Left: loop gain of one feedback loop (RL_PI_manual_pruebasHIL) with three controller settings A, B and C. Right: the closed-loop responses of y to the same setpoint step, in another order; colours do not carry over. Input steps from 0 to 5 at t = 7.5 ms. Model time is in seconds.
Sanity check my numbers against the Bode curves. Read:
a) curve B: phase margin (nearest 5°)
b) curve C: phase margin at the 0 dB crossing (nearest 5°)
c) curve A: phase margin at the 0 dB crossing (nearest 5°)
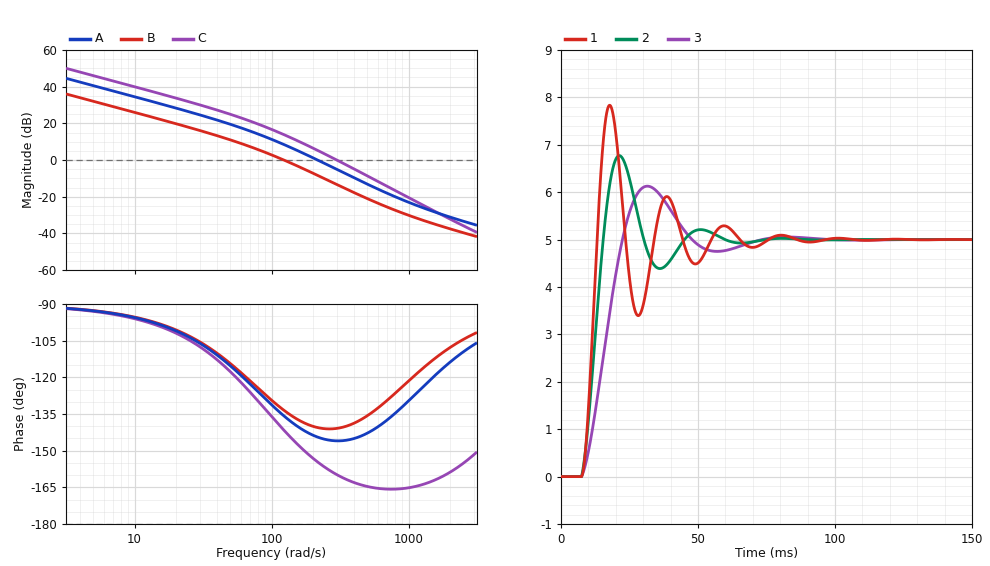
45°
20°
35°
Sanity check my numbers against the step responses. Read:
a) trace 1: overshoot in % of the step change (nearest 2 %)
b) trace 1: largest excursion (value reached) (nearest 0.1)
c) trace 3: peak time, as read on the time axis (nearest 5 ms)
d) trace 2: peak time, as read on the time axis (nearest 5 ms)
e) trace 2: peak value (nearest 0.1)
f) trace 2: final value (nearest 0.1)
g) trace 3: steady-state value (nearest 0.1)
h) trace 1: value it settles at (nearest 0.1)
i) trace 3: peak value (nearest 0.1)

56 %
7.8
30 ms
20 ms
6.8
5.0
5.0
5.0
6.1
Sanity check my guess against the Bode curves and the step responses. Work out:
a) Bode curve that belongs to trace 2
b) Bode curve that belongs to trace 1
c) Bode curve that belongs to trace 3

A
C
B
